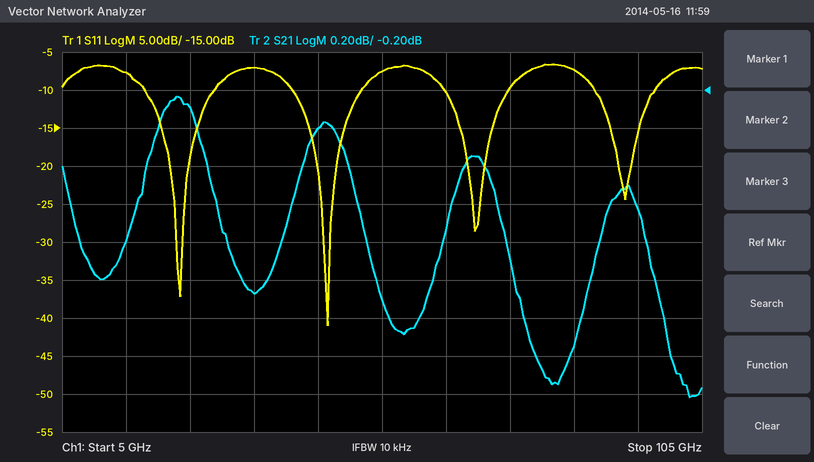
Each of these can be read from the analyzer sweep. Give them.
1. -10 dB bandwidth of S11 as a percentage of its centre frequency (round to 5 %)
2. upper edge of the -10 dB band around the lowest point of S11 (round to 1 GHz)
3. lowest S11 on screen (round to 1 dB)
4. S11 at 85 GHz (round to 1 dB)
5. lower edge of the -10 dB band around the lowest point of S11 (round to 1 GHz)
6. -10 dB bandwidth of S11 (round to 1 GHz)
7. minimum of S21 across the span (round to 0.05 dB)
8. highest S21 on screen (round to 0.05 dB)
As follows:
25 %
52 GHz
-41 dB
-7 dB
41 GHz
11 GHz
-1.80 dB
-0.25 dB
